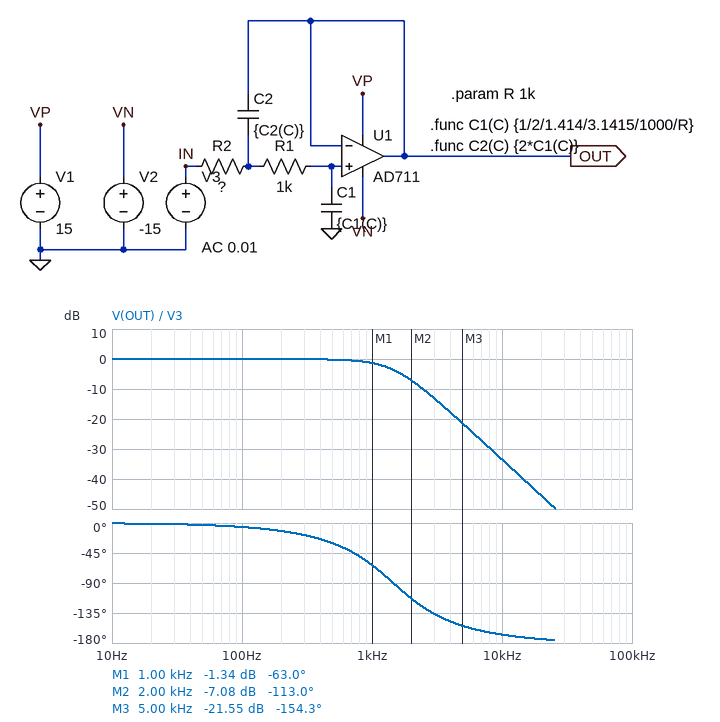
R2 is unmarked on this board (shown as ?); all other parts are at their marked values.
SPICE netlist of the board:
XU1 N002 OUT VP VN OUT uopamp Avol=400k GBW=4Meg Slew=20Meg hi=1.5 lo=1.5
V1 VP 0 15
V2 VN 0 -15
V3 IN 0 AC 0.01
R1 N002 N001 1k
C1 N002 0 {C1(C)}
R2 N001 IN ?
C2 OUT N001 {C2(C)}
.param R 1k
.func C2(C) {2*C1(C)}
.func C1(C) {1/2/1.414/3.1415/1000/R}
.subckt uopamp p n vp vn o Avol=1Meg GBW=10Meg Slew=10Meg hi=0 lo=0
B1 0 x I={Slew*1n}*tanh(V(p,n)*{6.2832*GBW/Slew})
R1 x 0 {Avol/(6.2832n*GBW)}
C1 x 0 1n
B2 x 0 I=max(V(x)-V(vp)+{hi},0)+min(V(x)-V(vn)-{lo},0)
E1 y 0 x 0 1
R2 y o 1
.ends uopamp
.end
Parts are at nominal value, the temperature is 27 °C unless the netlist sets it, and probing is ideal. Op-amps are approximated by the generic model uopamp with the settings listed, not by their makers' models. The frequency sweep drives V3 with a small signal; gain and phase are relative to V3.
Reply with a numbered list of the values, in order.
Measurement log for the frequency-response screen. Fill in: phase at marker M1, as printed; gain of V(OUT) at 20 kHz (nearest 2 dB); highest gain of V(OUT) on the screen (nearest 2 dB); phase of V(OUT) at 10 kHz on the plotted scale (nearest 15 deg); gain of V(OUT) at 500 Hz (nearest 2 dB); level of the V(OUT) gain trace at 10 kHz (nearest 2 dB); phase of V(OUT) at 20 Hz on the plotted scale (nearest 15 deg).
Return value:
1. -63.0 deg
2. -46 dB
3. 0 dB
4. -165 deg
5. 0 dB
6. -34 dB
7. 0 deg
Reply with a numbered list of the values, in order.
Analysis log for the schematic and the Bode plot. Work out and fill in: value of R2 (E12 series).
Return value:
1. 470 Ω
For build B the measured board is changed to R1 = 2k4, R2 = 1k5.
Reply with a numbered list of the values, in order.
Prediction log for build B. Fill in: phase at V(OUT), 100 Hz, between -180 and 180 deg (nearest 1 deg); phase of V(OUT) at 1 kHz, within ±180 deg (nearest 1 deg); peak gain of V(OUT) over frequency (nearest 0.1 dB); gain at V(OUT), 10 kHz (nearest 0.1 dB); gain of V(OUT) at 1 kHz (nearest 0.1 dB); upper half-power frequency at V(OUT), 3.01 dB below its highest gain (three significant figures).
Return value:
1. -16 deg
2. -133 deg
3. 0 dB
4. -51.1 dB
5. -11.6 dB
6. 512 Hz
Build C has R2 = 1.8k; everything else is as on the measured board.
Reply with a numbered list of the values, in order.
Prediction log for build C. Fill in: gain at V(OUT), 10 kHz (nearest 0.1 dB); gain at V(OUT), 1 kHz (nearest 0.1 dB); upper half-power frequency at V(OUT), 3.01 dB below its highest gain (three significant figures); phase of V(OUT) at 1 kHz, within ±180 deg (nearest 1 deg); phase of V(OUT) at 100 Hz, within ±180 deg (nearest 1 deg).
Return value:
1. -45.1 dB
2. -6.6 dB
3. 713 Hz
4. -112 deg
5. -11 deg
